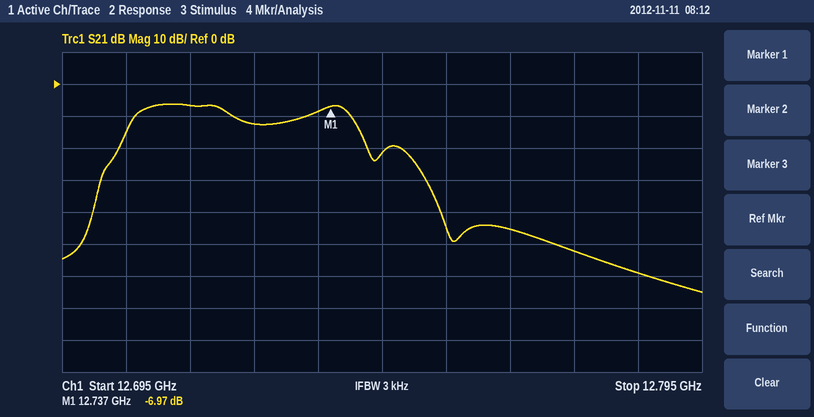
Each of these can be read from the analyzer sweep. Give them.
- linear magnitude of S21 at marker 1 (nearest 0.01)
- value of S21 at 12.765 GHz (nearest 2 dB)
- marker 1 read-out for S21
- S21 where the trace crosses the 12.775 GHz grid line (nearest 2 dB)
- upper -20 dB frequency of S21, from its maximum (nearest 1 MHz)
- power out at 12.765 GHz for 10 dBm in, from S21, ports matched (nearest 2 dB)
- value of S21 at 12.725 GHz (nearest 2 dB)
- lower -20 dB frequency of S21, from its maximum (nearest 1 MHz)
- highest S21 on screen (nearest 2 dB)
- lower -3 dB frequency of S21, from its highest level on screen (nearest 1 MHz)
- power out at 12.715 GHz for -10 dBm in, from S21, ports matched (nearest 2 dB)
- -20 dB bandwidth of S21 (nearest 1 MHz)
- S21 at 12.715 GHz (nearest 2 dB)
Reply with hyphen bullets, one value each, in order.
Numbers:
- 0.45
- -46 dB
- -6.97 dB
- -52 dB
- 12.751 GHz
- -36 dBm
- -12 dB
- 12.702 GHz
- -6 dB
- 12.707 GHz
- -16 dBm
- 49 MHz
- -6 dB
